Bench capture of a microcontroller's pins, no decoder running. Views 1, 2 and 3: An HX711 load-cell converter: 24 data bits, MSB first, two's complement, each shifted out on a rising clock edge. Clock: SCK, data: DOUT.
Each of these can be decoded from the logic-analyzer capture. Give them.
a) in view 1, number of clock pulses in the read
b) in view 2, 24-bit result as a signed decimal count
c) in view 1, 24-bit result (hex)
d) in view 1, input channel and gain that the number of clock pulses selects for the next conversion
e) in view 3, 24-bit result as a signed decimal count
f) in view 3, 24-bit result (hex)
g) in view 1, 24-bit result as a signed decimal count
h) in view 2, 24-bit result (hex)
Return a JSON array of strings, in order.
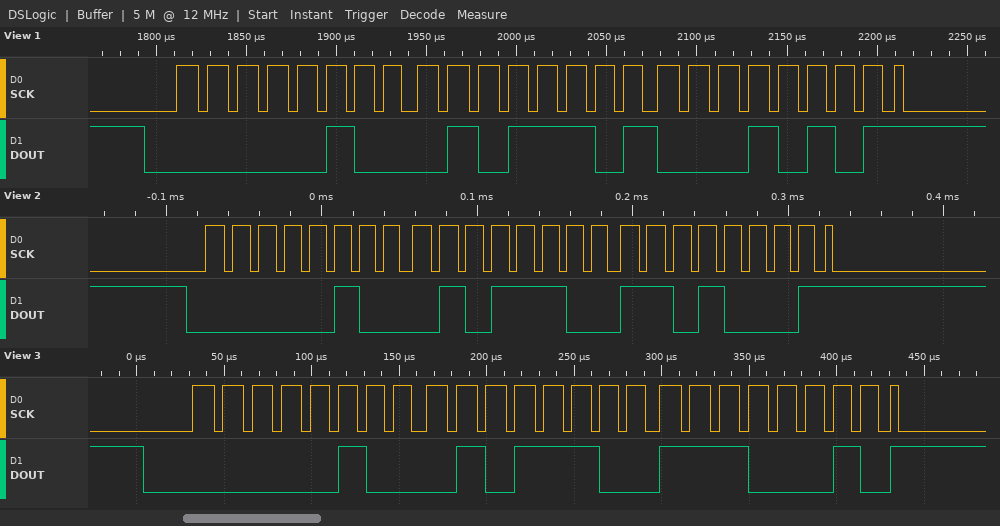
["25", "285905", "0x045D15", "channel A, gain 128", "285922", "0x045CE2", "285973", "0x045CD1"]
